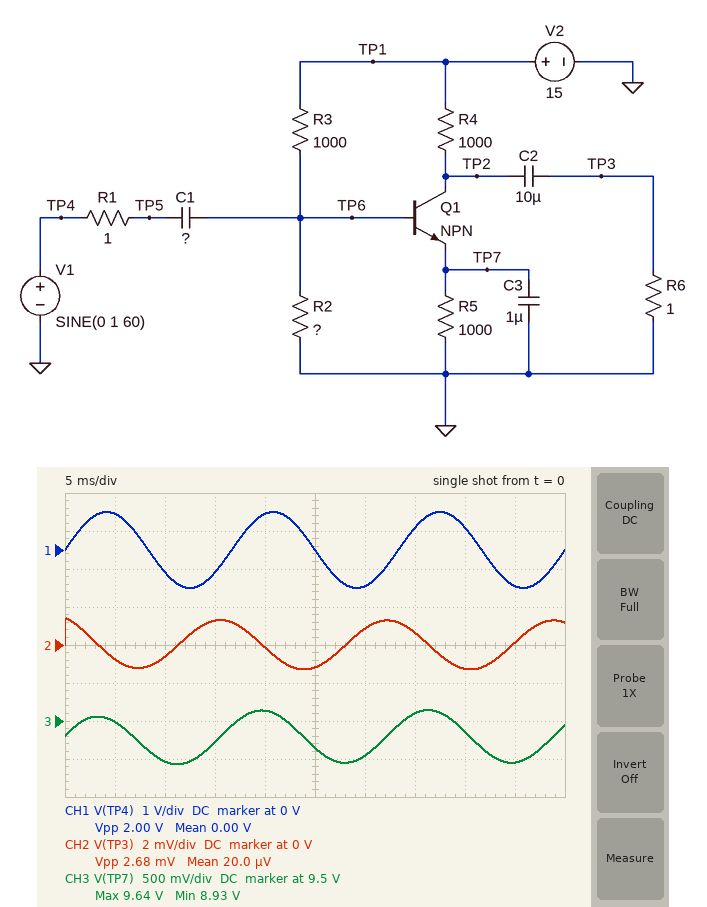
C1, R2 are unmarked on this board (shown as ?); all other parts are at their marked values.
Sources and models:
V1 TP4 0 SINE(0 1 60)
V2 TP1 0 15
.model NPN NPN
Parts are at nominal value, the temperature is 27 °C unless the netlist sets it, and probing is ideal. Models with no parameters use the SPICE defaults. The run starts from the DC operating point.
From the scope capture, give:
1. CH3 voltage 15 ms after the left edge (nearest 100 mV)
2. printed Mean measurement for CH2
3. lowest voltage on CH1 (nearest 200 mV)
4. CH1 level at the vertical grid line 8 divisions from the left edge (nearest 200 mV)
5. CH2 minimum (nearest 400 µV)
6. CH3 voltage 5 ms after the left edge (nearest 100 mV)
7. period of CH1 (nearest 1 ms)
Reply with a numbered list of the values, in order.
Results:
1. 9.2 V
2. 20.0 µV
3. -1.0 V
4. 600 mV
5. -1.2 mV
6. 9.5 V
7. 17 ms
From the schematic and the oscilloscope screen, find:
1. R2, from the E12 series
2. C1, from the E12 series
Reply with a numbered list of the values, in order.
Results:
1. 8.2 kΩ
2. 6.8 µF
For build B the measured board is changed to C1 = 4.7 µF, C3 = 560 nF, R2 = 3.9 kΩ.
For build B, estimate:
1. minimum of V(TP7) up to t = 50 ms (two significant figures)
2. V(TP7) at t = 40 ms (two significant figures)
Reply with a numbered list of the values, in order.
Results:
1. 8.6 V
2. 8.9 V
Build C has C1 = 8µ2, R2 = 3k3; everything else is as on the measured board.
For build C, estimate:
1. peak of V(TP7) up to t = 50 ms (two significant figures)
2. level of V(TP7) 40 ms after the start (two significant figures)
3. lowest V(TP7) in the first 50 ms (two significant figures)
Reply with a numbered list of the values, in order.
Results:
1. 9.1 V
2. 8.8 V
3. 8.3 V
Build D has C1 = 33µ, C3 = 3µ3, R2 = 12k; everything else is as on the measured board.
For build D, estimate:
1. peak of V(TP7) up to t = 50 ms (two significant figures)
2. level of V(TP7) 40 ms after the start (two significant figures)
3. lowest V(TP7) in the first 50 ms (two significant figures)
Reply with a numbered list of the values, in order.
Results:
1. 10 V
2. 9.7 V
3. 8.7 V
